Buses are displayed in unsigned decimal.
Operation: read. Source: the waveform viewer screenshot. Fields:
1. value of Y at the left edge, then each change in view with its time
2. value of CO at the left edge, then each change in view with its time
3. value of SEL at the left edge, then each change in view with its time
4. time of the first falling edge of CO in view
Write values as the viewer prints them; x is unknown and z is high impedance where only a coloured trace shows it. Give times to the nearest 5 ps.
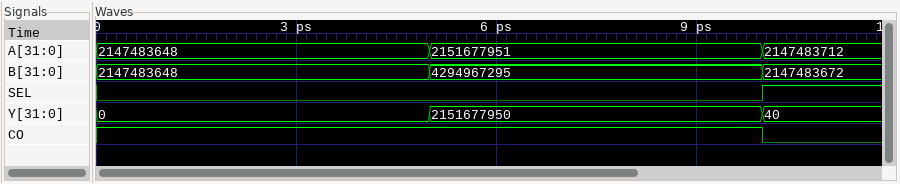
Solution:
0, 2151677950 at 5 ps, 40 at 10 ps
1, 0 at 10 ps
0, 1 at 10 ps
10 ps
